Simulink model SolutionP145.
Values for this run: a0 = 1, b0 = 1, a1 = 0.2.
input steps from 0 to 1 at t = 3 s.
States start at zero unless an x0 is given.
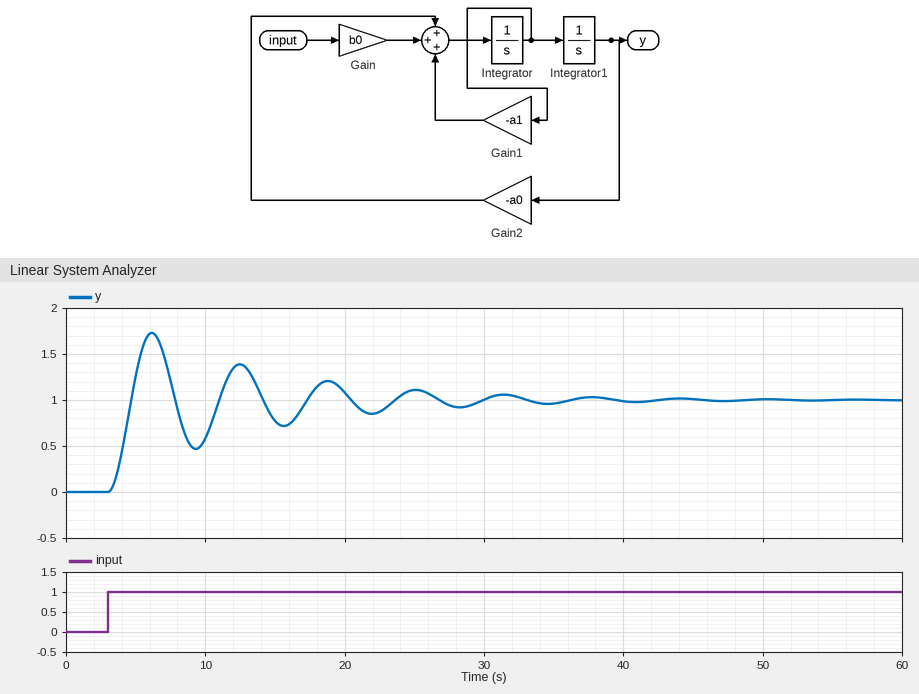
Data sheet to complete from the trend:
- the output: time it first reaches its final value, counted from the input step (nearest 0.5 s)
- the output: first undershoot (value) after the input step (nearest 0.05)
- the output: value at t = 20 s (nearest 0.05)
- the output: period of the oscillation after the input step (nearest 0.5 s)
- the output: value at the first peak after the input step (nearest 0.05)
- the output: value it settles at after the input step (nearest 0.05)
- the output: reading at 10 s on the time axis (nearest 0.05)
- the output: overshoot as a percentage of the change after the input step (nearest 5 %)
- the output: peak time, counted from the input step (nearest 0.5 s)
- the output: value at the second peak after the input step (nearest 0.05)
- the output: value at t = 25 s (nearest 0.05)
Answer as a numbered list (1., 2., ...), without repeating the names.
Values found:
1. 1.5 s
2. 0.45
3. 1.10
4. 6.5 s
5. 1.75
6. 1.00
7. 0.60
8. 75 %
9. 3.0 s
10. 1.40
11. 1.10
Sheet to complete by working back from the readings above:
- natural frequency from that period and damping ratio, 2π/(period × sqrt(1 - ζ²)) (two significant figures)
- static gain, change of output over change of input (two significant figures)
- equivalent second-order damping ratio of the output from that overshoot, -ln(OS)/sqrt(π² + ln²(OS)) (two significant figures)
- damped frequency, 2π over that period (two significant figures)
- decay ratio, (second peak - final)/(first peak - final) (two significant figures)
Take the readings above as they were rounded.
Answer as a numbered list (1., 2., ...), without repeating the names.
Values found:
1. 0.97 rad/s
2. 1.0
3. 0.091
4. 0.97 rad/s
5. 0.53
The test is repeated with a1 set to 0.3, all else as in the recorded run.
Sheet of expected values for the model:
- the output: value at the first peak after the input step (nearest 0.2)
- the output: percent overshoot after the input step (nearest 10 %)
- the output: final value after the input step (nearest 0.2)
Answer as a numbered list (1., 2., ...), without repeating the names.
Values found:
1. 1.6
2. 60 %
3. 1.0
